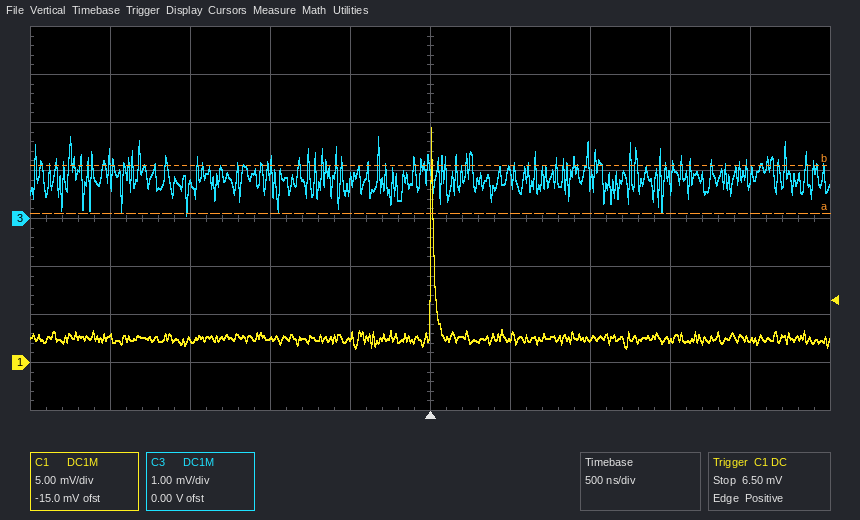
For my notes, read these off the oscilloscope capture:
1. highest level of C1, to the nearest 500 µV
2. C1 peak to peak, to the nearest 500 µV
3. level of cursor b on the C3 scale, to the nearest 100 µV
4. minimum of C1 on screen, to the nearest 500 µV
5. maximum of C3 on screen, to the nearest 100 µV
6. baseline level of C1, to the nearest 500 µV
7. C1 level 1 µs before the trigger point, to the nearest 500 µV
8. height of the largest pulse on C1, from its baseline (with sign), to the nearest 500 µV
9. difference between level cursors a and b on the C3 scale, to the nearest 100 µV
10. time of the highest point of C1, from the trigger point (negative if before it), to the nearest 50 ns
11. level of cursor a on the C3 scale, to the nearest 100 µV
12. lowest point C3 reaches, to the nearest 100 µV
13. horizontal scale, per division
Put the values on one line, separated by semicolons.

24.5 mV; 23.0 mV; 1.1 mV; 1.5 mV; 1.7 mV; 2.5 mV; 2.5 mV; +22.0 mV; 1.0 mV; 0 ns; 100 µV; 100 µV; 500 ns
